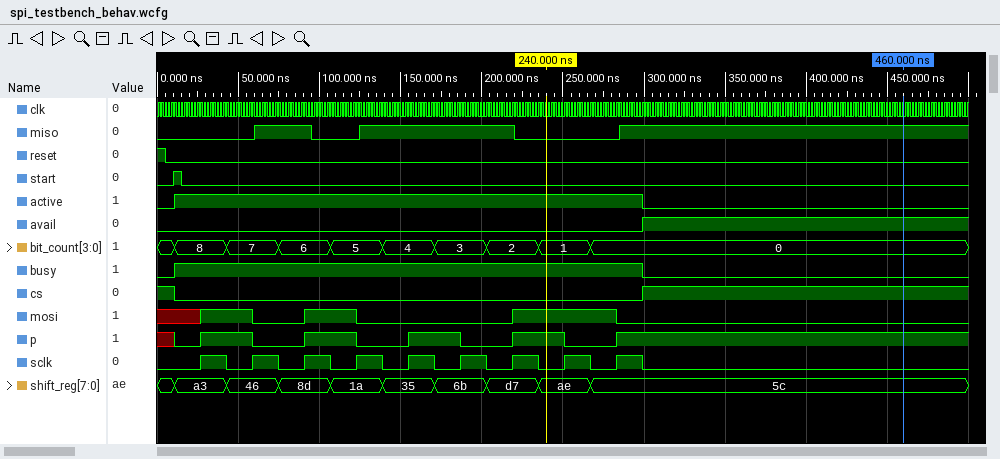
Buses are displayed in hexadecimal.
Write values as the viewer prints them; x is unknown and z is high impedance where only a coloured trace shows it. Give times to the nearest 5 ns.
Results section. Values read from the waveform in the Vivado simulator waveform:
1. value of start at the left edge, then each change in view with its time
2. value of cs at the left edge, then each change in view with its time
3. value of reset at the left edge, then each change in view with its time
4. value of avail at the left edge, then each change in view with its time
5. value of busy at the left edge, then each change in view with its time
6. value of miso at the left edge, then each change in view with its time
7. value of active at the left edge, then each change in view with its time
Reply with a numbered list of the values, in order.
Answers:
1. 0, 1 at 10 ns, 0 at 15 ns
2. 1, 0 at 10 ns, 1 at 300 ns
3. 1, 0 at 5 ns
4. 0, 1 at 300 ns
5. 0, 1 at 10 ns, 0 at 300 ns
6. 0, 1 at 60 ns, 0 at 95 ns, 1 at 125 ns, 0 at 220 ns, 1 at 285 ns
7. 0, 1 at 10 ns, 0 at 300 ns
